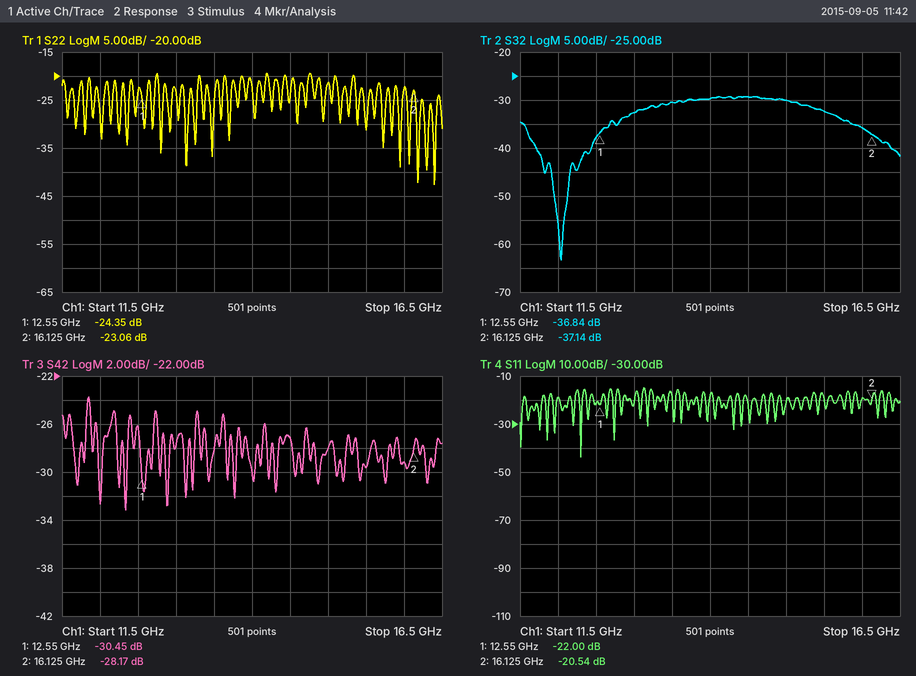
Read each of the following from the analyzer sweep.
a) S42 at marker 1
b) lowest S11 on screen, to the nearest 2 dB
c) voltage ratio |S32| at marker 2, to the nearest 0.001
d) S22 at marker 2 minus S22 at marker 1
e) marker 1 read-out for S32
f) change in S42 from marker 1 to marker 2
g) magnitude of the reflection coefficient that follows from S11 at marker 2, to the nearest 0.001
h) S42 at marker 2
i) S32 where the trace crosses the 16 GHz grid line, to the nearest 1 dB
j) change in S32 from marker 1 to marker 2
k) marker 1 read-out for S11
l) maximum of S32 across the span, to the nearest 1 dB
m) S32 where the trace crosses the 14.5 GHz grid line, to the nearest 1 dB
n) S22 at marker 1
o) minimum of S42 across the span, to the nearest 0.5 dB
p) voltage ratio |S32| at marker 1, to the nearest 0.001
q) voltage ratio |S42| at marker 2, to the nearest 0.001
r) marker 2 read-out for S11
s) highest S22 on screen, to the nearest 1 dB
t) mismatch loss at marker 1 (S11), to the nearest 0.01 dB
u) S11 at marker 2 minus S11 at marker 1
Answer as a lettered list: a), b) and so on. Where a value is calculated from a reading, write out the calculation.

a) -30.45 dB
b) -44 dB
c) 10^(-37.14/20) ≈ 0.014
d) -23.06 − (-24.35) = 1.29 dB
e) -36.84 dB
f) -28.17 − (-30.45) = 2.28 dB
g) 10^(-20.54/20) ≈ 0.094
h) -28.17 dB
i) -36 dB
j) -37.14 − (-36.84) = -0.30 dB
k) -22.00 dB
l) -29 dB
m) -29 dB
n) -24.35 dB
o) -33.0 dB
p) 10^(-36.84/20) ≈ 0.014
q) 10^(-28.17/20) ≈ 0.039
r) -20.54 dB
s) -19 dB
t) −10 log10(1 − 10^(-22/10)) ≈ 0.03 dB
u) -20.54 − (-22) = 1.46 dB
